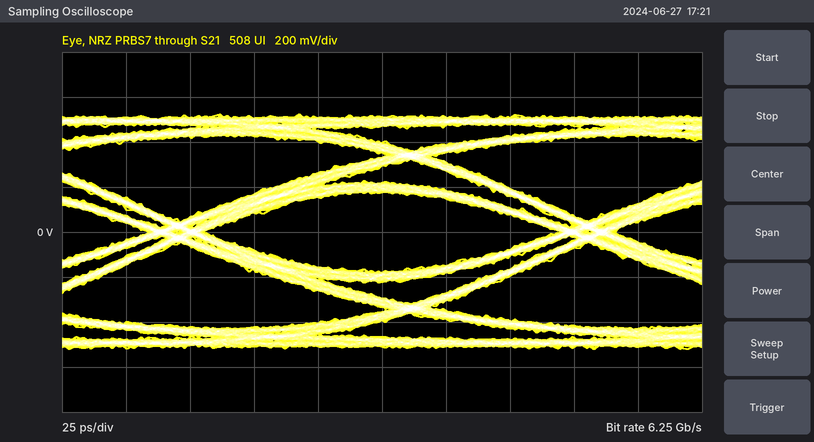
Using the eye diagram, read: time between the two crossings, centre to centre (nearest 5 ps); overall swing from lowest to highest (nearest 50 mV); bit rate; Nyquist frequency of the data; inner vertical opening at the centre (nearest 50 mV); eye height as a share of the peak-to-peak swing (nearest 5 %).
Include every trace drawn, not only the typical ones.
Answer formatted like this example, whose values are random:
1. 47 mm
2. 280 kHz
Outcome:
1. 160 ps
2. 1.05 V
3. 6.25 Gb/s
4. 3.125 GHz
5. 350 mV
6. 35 %
